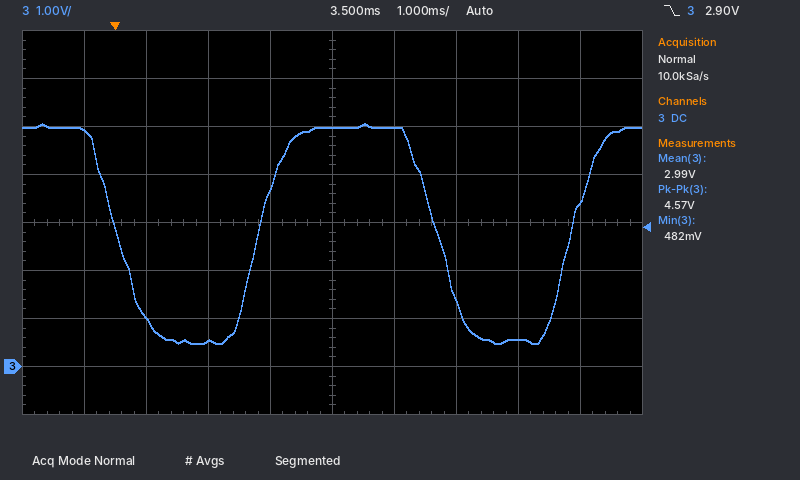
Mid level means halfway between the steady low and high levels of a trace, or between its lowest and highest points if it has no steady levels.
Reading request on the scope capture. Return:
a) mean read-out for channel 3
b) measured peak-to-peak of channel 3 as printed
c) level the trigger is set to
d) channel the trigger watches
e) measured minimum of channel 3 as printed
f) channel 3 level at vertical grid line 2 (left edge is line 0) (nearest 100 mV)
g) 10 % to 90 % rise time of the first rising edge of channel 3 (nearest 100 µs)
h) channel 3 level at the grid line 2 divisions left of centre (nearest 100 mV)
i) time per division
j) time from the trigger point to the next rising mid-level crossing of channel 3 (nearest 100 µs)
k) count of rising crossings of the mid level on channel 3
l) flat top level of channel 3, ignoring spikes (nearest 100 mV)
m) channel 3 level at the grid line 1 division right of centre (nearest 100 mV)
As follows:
2.99 V
4.57 V
2.90 V
channel 3
482 mV
1.0 V
800 µs
500 mV
1 ms
2.3 ms
2
5.0 V
5.0 V
